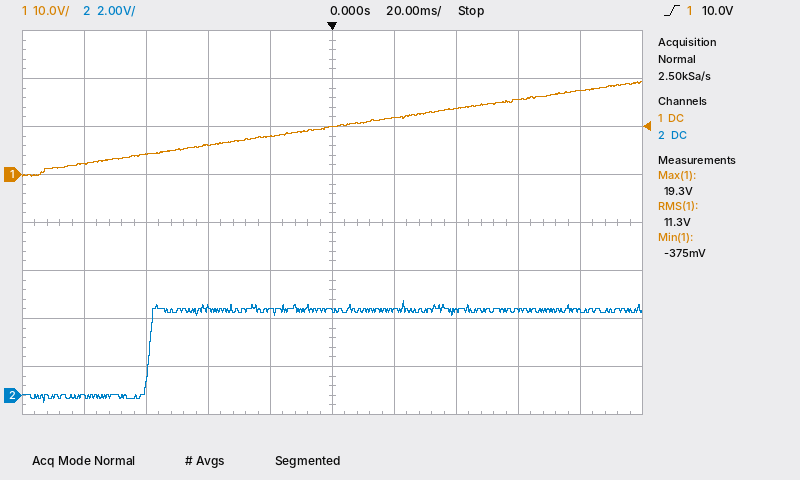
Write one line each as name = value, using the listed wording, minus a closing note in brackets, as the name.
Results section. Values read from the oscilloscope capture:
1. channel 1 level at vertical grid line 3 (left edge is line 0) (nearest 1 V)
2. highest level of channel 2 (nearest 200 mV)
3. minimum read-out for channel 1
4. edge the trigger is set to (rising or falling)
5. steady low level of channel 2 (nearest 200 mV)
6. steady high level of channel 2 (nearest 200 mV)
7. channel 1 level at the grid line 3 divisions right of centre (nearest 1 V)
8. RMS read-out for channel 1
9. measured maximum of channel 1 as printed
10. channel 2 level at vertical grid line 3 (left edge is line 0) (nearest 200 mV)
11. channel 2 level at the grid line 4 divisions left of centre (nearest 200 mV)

channel 1 level at vertical grid line 3 (left edge is line 0) = 6 V
highest level of channel 2 = 4.0 V
minimum read-out for channel 1 = -375 mV
edge the trigger is set to = rising
steady low level of channel 2 = 0.0 V
steady high level of channel 2 = 3.6 V
channel 1 level at the grid line 3 divisions right of centre = 16 V
RMS read-out for channel 1 = 11.3 V
measured maximum of channel 1 as printed = 19.3 V
channel 2 level at vertical grid line 3 (left edge is line 0) = 3.6 V
channel 2 level at the grid line 4 divisions left of centre = 0.0 V
